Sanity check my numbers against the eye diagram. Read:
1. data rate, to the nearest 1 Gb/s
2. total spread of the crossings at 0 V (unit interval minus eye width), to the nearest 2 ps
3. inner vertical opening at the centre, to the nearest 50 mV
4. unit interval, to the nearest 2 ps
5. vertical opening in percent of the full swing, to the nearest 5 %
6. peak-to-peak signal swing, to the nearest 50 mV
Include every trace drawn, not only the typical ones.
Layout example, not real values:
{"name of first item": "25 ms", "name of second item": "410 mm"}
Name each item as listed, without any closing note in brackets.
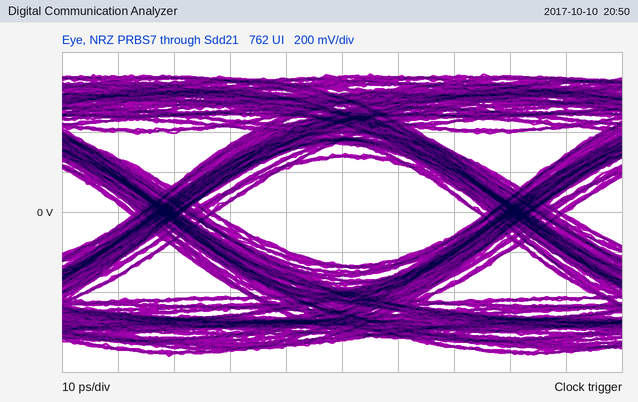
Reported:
{"data rate, to the nearest 1 Gb/s": "16 Gb/s", "total spread of the crossings at 0 V (unit interval minus eye width), to the nearest 2 ps": "16 ps", "inner vertical opening at the centre, to the nearest 50 mV": "550 mV", "unit interval, to the nearest 2 ps": "62 ps", "vertical opening in percent of the full swing, to the nearest 5 %": "40 %", "peak-to-peak signal swing, to the nearest 50 mV": "1.40 V"}
